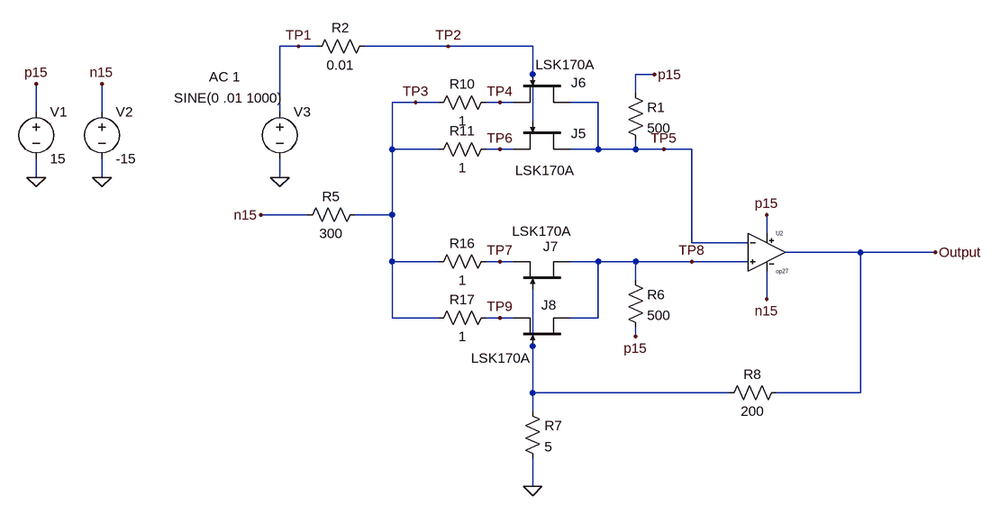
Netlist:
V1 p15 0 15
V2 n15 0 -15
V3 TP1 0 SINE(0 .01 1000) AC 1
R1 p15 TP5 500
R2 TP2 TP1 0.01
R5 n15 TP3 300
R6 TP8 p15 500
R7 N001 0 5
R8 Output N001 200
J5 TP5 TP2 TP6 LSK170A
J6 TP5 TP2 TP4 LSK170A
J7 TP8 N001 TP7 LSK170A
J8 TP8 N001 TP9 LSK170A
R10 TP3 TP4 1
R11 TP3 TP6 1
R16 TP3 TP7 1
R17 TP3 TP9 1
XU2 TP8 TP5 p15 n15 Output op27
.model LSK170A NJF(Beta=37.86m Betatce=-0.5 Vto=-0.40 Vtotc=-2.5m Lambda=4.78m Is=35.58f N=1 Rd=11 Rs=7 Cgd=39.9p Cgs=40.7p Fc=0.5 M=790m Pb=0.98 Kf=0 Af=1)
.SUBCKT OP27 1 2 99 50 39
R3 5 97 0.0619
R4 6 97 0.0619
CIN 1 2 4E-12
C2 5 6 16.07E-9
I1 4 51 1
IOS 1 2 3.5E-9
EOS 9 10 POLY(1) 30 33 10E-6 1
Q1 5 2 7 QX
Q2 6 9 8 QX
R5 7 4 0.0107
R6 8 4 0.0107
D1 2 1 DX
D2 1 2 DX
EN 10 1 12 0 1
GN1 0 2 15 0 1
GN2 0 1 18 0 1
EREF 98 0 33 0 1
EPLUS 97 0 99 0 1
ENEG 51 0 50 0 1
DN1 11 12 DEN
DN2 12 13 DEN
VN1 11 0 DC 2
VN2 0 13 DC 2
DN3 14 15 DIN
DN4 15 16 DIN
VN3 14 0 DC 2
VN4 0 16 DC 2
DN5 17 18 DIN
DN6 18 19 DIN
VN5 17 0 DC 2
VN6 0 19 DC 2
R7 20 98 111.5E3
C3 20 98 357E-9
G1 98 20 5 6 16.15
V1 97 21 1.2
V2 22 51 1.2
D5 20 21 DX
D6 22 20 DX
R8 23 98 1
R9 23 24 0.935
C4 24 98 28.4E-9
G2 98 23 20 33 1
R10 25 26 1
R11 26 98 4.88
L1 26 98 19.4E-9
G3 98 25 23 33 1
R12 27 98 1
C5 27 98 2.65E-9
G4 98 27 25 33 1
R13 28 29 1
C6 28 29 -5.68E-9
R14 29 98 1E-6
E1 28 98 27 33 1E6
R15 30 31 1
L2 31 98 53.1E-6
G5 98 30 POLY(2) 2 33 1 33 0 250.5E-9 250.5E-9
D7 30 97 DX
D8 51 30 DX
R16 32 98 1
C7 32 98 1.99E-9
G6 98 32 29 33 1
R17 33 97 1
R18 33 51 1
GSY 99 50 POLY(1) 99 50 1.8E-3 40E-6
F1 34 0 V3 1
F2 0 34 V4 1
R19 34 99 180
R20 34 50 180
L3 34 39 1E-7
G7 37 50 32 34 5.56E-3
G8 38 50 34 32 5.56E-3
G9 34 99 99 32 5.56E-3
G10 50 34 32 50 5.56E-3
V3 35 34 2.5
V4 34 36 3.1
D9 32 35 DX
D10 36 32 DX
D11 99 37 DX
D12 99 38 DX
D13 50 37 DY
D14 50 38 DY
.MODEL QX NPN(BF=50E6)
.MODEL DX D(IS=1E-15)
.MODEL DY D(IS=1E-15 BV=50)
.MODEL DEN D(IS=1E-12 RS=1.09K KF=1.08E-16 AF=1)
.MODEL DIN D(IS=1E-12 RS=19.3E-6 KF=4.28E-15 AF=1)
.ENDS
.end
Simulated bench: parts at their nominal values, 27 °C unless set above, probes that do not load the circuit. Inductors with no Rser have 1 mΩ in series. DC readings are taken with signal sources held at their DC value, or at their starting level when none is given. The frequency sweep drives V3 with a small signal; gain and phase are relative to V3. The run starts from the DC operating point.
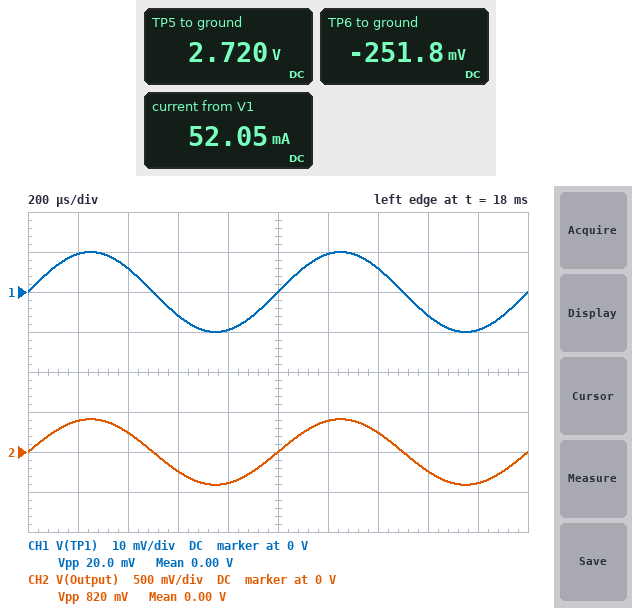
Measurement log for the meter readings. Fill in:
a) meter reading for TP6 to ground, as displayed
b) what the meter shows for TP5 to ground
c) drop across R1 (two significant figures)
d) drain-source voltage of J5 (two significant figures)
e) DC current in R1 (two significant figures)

-251.8 mV
2.720 V
12 V
3.0 V
25 mA
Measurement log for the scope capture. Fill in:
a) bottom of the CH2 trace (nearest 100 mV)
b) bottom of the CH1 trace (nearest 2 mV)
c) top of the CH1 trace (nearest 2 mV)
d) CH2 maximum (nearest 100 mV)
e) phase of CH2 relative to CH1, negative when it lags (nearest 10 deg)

-400 mV
-10 mV
10 mV
400 mV
0 deg
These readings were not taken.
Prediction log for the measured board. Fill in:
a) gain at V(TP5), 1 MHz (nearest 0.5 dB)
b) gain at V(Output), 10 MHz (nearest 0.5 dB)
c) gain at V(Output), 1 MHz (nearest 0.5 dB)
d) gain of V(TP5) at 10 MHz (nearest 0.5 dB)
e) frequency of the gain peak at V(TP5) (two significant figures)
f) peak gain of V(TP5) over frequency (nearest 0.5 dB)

12.5 dB
19.0 dB
32.5 dB
20.0 dB
3.9 MHz
25.5 dB
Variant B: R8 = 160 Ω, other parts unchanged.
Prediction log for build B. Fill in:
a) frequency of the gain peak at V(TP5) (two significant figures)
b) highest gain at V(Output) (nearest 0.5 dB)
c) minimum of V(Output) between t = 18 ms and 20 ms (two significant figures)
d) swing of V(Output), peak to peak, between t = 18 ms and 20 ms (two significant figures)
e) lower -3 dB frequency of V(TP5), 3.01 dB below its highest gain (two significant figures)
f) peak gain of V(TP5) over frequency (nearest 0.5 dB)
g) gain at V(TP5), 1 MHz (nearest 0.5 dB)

4.2 MHz
32.5 dB
-330 mV
660 mV
2.7 MHz
26.0 dB
11.5 dB
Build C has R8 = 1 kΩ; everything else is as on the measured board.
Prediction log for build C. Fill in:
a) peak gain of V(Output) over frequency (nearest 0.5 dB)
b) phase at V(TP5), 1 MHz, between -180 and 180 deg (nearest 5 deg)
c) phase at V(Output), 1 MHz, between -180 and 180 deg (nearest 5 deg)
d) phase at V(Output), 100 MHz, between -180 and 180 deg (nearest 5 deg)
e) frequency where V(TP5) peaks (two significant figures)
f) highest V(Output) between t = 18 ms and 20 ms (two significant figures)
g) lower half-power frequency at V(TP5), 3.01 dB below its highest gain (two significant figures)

46.0 dB
-140 deg
-55 deg
-75 deg
2.1 MHz
2.0 V
900 kHz
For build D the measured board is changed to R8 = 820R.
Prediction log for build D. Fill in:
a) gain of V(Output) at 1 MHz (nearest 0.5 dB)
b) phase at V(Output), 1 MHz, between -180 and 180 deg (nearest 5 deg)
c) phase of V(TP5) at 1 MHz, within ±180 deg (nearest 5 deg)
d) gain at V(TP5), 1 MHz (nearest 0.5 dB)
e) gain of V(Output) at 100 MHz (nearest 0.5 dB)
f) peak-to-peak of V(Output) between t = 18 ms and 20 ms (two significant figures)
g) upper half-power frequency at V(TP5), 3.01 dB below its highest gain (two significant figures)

43.5 dB
-50 deg
-135 deg
21.5 dB
-12.5 dB
3.3 V
6.0 MHz
